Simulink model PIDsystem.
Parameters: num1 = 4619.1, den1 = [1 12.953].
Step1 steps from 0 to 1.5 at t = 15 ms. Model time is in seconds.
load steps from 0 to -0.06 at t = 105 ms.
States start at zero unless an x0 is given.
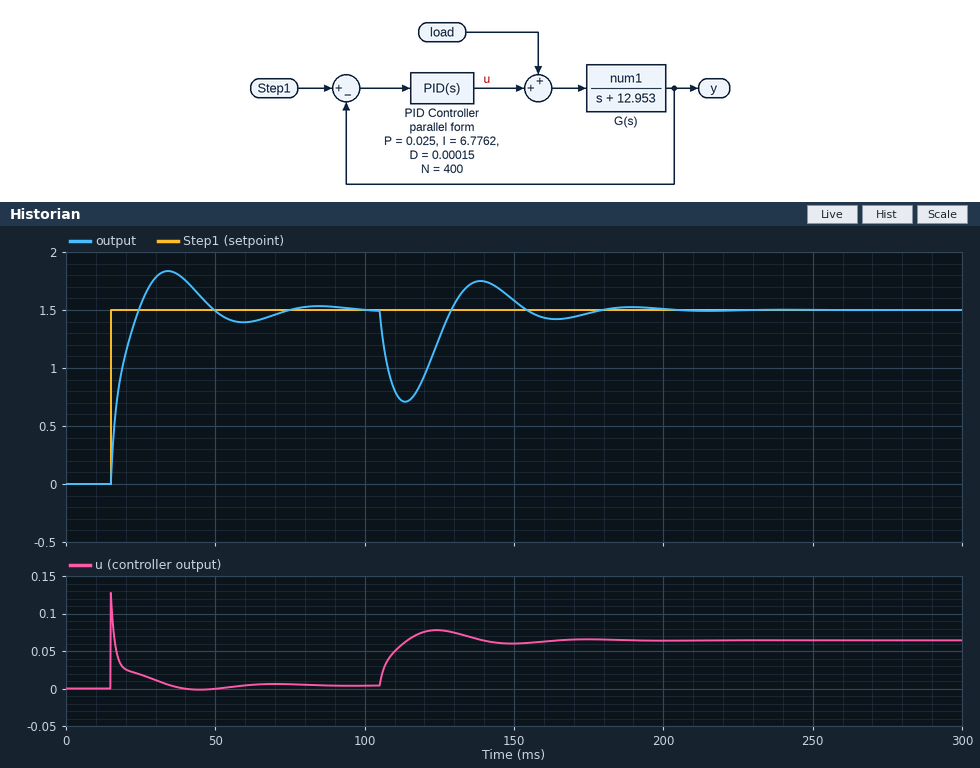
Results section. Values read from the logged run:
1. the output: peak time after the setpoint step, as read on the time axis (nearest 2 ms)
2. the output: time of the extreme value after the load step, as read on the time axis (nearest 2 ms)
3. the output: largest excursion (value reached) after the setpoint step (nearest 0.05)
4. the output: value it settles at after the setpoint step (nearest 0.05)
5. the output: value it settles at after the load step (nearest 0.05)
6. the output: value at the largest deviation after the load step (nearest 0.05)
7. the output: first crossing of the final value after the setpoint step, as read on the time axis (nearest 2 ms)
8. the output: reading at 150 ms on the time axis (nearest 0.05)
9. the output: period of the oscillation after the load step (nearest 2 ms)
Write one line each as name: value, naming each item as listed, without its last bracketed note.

the output: peak time after the setpoint step, as read on the time axis: 34 ms
the output: time of the extreme value after the load step, as read on the time axis: 114 ms
the output: largest excursion (value reached) after the setpoint step: 1.85
the output: value it settles at after the setpoint step: 1.50
the output: value it settles at after the load step: 1.50
the output: value at the largest deviation after the load step: 0.70
the output: first crossing of the final value after the setpoint step, as read on the time axis: 24 ms
the output: reading at 150 ms on the time axis: 1.60
the output: period of the oscillation after the load step: 50 ms
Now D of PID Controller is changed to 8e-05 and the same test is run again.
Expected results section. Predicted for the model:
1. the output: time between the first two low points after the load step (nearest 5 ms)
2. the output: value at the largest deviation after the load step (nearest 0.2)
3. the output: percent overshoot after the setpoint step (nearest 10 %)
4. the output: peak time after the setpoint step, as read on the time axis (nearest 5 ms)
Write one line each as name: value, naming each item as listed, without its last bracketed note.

the output: time between the first two low points after the load step: 45 ms
the output: value at the largest deviation after the load step: 0.6
the output: percent overshoot after the setpoint step: 30 %
the output: peak time after the setpoint step, as read on the time axis: 30 ms
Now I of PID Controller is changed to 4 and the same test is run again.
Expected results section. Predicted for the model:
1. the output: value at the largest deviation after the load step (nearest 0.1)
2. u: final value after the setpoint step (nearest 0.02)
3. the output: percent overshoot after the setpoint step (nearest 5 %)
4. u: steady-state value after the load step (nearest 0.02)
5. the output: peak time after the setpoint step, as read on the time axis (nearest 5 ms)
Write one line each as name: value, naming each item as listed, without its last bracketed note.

the output: value at the largest deviation after the load step: 0.6
u: final value after the setpoint step: 0.00
the output: percent overshoot after the setpoint step: 20 %
u: steady-state value after the load step: 0.06
the output: peak time after the setpoint step, as read on the time axis: 40 ms
